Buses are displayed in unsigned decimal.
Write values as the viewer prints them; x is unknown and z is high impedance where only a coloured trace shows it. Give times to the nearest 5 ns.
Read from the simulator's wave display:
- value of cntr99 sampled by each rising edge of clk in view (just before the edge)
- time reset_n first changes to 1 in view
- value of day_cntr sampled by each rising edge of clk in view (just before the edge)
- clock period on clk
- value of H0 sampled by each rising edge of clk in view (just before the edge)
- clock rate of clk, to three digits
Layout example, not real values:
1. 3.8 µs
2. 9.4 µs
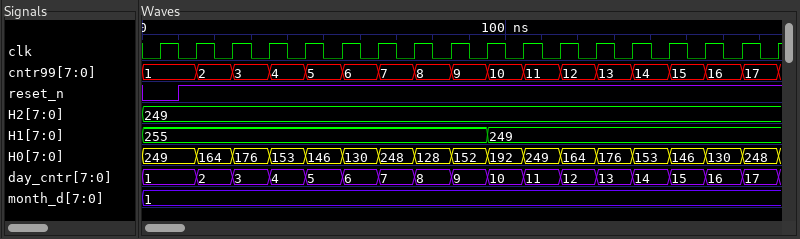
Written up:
1. 1, 1, 2, 3, 4, 5, 6, 7, 8, 9, 10, 11, 12, 13, 14, 15, 16, 17
2. 10 ns
3. 1, 1, 2, 3, 4, 5, 6, 7, 8, 9, 10, 11, 12, 13, 14, 15, 16, 17
4. 10 ns
5. 249, 249, 164, 176, 153, 146, 130, 248, 128, 152, 192, 249, 164, 176, 153, 146, 130, 248
6. 100 MHz
